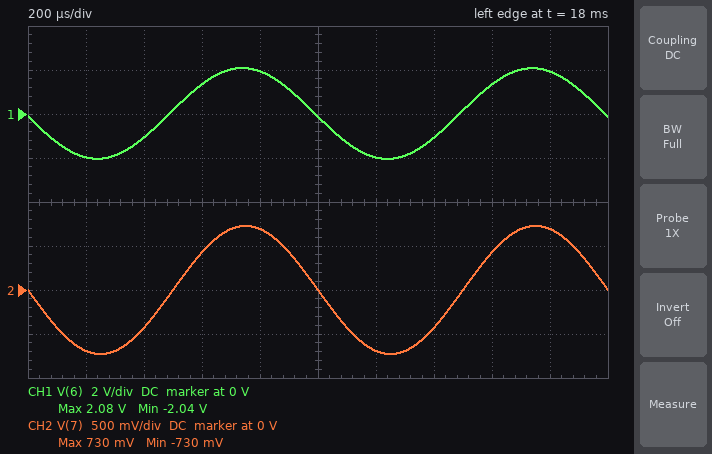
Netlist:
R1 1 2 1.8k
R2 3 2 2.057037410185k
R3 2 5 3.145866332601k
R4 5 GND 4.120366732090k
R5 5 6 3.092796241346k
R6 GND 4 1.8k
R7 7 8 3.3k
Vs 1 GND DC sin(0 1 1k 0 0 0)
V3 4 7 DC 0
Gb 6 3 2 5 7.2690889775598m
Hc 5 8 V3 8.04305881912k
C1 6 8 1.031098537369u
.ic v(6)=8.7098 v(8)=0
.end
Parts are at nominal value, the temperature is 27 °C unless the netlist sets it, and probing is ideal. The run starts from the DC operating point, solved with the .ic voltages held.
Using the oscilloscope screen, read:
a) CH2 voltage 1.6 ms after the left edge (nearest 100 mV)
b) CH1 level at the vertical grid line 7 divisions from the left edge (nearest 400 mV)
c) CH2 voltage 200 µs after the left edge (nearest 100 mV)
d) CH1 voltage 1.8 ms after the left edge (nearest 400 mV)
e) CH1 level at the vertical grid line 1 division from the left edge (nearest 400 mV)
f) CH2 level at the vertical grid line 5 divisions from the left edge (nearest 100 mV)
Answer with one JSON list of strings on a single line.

["400 mV", "-1.2 V", "-700 mV", "2.0 V", "-2.0 V", "0 V"]
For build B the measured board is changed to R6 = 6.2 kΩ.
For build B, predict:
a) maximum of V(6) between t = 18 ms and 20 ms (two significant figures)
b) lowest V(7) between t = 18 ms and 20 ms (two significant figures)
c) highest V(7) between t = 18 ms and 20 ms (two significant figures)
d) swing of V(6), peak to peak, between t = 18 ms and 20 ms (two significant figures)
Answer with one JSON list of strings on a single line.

["2.6 V", "-1.7 V", "1.7 V", "5.1 V"]
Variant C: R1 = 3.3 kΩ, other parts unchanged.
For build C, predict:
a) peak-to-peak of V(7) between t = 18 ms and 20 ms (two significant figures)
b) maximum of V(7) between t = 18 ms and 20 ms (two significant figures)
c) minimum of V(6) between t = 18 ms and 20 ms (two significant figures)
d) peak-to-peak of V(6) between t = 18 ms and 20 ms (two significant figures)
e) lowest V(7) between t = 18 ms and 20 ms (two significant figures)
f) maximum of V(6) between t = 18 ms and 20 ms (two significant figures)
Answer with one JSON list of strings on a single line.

["1.8 V", "880 mV", "-2.5 V", "5.0 V", "-880 mV", "2.5 V"]
